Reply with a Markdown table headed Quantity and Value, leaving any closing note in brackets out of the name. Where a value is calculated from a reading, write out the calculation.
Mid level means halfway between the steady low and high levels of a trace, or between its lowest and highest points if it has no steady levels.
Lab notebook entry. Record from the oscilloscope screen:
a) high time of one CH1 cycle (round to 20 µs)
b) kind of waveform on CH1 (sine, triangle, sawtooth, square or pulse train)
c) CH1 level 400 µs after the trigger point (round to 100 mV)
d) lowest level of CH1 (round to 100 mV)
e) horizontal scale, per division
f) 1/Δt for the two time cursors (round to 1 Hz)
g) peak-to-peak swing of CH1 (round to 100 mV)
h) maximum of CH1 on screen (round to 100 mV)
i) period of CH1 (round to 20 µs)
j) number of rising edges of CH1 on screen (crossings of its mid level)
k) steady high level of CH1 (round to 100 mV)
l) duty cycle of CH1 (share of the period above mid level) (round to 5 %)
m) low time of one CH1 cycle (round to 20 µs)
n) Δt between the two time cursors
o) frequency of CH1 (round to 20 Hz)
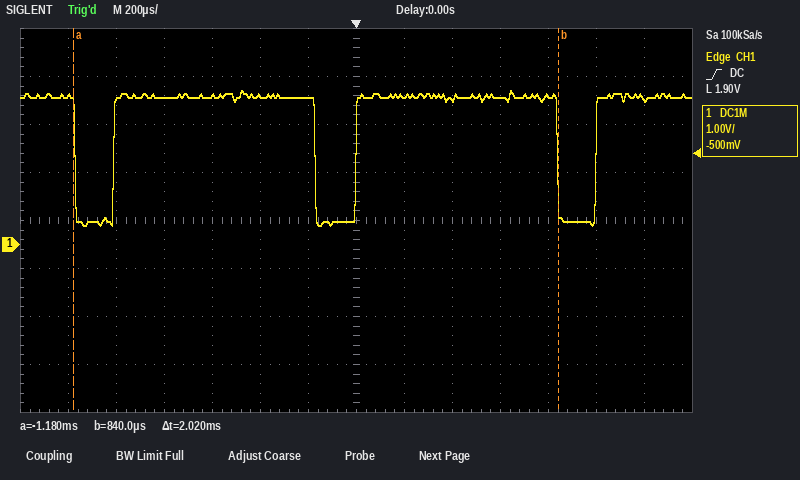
| Quantity | Value |
|---|---|
| high time of one CH1 cycle | 840 µs |
| kind of waveform on CH1 | pulse train |
| CH1 level 400 µs after the trigger point | 3.0 V |
| lowest level of CH1 | 400 mV |
| horizontal scale, per division | 200 µs |
| 1/Δt for the two time cursors | 1 / 2.02 ms ≈ 495 Hz |
| peak-to-peak swing of CH1 | 3.2 V − (400 mV) = 2.8 V |
| maximum of CH1 on screen | 3.2 V |
| period of CH1 | 1.00 ms |
| number of rising edges of CH1 on screen | 3 |
| steady high level of CH1 | 3.1 V |
| duty cycle of CH1 (share of the period above mid level) | 840 µs / 1.00 ms ≈ 84.0 %, so 85 % to the nearest 5 % |
| low time of one CH1 cycle | 160 µs |
| Δt between the two time cursors | 2.02 ms |
| frequency of CH1 | 1 / 1.00 ms ≈ 1.00 kHz |
